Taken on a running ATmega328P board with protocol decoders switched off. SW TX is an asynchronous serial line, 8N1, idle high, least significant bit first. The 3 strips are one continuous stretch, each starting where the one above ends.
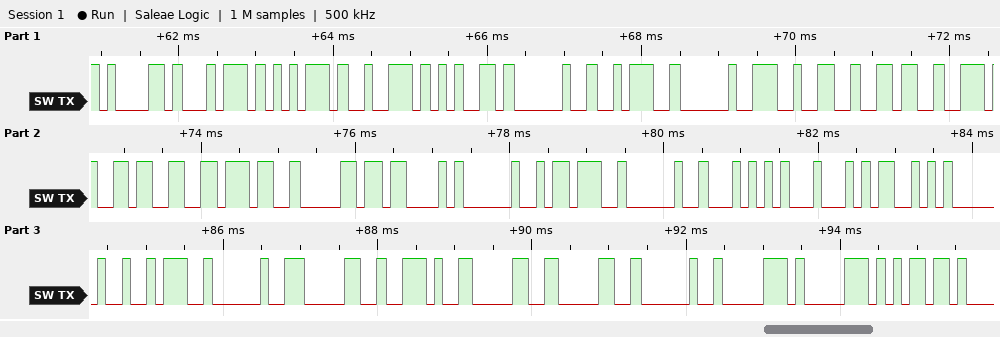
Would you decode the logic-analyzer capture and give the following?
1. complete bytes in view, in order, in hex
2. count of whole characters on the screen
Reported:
0x61 0x74 0x75 0x72 0x65 0x20 0x3A 0x20 0x32 0x36 0x2E 0x33 0x37 0xB0 0x43 0x20 0x3B 0x20 0x54 0x44 0x53 0x20 0x3A 0x20 0x30 0x2E 0x30 0x30 0x20 0x70 0x70 0x6D
32
